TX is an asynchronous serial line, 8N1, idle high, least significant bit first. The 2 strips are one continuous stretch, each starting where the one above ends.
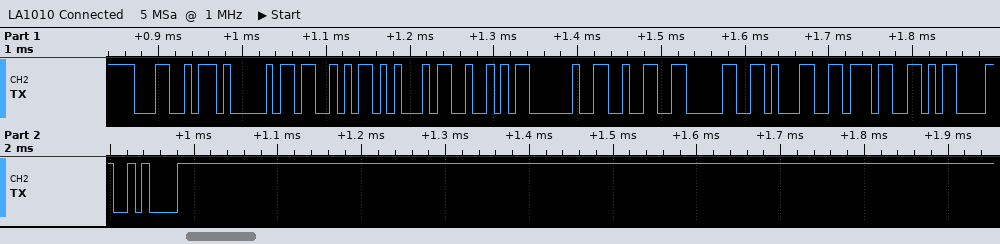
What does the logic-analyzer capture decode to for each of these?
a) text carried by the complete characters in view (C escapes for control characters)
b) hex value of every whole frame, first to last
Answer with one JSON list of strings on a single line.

["\"LASER 2017\\r\\n\"", "4C 41 53 45 52 20 32 30 31 37 0D 0A"]
